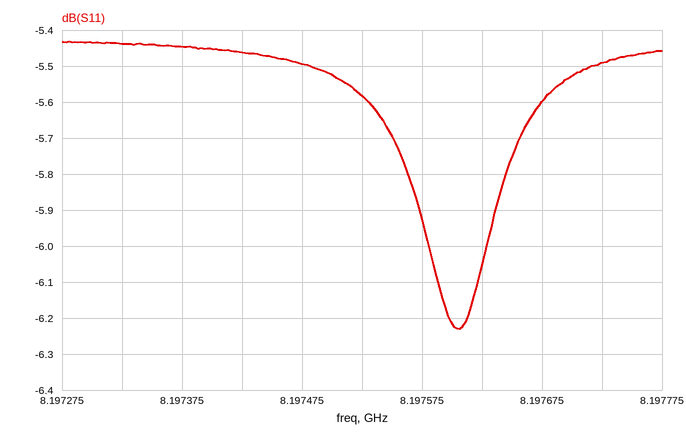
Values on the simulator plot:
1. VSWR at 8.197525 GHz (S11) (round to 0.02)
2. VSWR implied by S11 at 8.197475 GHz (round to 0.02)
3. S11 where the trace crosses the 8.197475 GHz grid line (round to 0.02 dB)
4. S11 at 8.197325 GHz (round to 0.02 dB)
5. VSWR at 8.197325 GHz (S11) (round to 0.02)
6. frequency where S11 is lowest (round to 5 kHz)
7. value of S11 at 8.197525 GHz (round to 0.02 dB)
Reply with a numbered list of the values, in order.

1. 3.22
2. 3.26
3. -5.50 dB
4. -5.44 dB
5. 3.30
6. 8.197605 GHz
7. -5.58 dB
